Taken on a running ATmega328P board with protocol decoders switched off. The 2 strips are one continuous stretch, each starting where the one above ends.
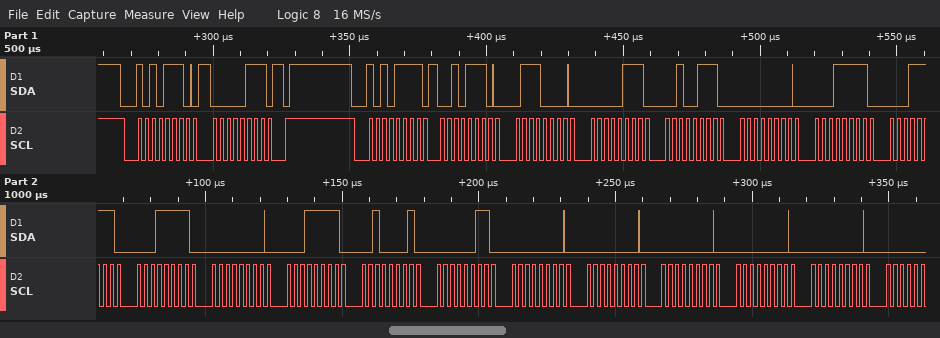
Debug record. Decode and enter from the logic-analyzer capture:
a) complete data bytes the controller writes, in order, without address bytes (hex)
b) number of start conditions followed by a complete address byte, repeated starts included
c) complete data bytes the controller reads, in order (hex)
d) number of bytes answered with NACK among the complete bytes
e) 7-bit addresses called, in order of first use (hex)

07
2
2E 70 07 27 00 1F 1F 1F 00 1F 21 03 00 00 00 00 00
0
0x57
